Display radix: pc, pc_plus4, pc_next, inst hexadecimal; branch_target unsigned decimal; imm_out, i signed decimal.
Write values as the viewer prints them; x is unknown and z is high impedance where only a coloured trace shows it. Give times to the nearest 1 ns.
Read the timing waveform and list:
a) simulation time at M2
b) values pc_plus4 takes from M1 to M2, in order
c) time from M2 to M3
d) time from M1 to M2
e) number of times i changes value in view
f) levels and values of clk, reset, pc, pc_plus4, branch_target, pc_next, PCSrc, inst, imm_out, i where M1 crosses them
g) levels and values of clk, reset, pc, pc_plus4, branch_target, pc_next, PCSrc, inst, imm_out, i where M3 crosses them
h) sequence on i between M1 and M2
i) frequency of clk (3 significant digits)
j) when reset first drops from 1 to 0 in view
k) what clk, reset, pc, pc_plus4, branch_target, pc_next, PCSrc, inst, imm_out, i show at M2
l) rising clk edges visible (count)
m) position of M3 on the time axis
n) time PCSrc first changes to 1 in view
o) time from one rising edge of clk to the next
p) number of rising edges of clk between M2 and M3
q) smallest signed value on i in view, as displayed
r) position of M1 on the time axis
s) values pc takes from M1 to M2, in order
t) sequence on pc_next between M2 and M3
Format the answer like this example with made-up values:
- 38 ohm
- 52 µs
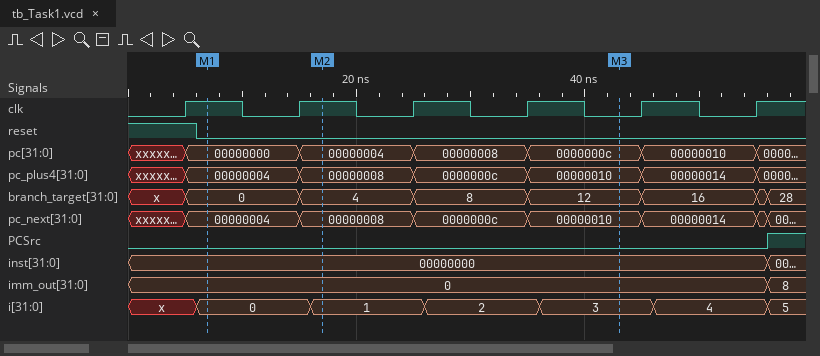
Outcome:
- 17 ns
- 00000004, 00000008
- 26 ns
- 10 ns
- 6
- clk=1, reset=0, pc=00000000, pc_plus4=00000004, branch_target=0, pc_next=00000004, PCSrc=0, inst=00000000, imm_out=0, i=0
- clk=0, reset=0, pc=0000000c, pc_plus4=00000010, branch_target=12, pc_next=00000010, PCSrc=0, inst=00000000, imm_out=0, i=3
- 0, 1
- 100 MHz
- 6 ns
- clk=1, reset=0, pc=00000004, pc_plus4=00000008, branch_target=4, pc_next=00000008, PCSrc=0, inst=00000000, imm_out=0, i=1
- 6
- 43 ns
- 56 ns
- 10 ns
- 2
- 0
- 7 ns
- 00000000, 00000004
- 00000008, 0000000c, 00000010
